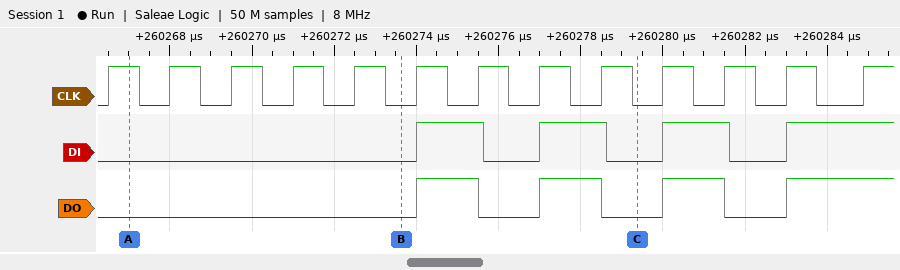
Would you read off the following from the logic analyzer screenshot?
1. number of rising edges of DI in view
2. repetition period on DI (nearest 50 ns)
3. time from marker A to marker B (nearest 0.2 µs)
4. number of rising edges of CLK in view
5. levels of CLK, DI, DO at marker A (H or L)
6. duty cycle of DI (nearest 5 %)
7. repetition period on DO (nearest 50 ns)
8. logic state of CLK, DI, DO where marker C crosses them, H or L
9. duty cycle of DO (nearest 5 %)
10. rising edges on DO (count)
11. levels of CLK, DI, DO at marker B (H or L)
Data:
4
3000 ns
6.6 µs
13
CLK=H, DI=L, DO=L
55 %
3000 ns
CLK=L, DI=L, DO=L
50 %
4
CLK=L, DI=L, DO=L
